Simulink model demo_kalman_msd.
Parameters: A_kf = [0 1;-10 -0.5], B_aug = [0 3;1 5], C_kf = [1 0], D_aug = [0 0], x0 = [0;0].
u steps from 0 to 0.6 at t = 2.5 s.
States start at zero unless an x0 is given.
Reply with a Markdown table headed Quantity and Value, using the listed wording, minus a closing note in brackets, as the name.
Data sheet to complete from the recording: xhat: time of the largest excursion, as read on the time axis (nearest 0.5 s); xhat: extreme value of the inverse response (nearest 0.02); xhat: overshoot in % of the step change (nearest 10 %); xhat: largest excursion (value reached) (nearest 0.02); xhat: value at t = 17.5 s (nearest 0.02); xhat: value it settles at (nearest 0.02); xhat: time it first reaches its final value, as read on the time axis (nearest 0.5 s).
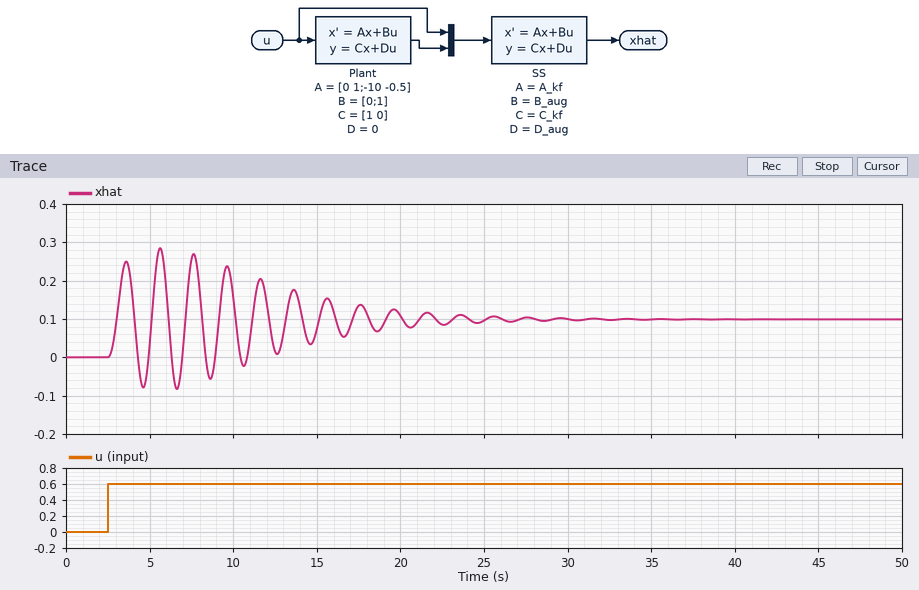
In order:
| Quantity | Value |
|---|---|
| xhat: time of the largest excursion, as read on the time axis | 5.5 s |
| xhat: extreme value of the inverse response | -0.08 |
| xhat: overshoot in % of the step change | 190 % |
| xhat: largest excursion (value reached) | 0.28 |
| xhat: value at t = 17.5 s | 0.14 |
| xhat: value it settles at | 0.10 |
| xhat: time it first reaches its final value, as read on the time axis | 3.0 s |
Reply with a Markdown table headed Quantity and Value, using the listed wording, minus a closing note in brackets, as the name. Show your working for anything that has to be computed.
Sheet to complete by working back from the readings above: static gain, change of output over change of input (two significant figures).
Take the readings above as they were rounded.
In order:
| Quantity | Value |
|---|---|
| static gain, change of output over change of input | (0.1 - 0) / (0.6 - 0) = 0.17 |
